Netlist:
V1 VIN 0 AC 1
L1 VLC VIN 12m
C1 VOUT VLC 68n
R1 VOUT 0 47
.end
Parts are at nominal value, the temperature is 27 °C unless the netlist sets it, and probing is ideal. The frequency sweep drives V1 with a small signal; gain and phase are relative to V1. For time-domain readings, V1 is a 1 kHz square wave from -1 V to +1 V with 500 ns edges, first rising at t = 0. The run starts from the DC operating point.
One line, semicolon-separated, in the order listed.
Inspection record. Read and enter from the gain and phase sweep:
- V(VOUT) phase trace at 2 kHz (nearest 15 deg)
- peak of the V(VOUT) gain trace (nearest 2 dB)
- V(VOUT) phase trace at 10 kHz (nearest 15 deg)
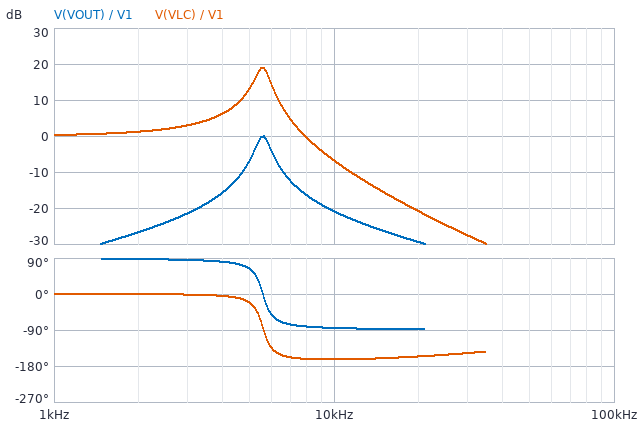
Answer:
90 deg; 0 dB; -90 deg
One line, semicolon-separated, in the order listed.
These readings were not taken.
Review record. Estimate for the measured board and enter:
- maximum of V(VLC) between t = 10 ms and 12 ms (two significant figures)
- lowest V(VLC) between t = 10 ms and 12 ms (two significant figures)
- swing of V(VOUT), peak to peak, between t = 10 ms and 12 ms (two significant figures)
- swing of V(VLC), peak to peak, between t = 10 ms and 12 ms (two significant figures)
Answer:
2.5 V; -2.5 V; 370 mV; 5.0 V
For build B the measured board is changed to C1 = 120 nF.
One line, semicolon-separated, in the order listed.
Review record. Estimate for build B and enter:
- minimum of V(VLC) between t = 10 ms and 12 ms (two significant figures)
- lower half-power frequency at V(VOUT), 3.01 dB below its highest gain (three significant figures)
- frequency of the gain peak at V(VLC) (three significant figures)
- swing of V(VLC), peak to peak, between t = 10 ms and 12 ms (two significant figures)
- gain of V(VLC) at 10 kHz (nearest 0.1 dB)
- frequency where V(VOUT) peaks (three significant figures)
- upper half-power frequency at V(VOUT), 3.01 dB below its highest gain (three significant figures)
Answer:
-2.2 V; 3.89 kHz; 4.17 kHz; 4.4 V; -12.9 dB; 4.19 kHz; 4.52 kHz
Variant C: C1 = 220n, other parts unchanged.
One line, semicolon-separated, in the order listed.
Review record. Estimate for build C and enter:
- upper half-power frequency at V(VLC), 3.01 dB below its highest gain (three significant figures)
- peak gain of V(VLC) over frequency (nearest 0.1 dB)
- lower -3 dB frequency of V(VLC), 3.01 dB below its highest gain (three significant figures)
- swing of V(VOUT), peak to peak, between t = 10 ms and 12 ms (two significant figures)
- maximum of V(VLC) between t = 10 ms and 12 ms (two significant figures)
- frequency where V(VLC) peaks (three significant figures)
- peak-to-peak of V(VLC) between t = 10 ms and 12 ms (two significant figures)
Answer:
3.37 kHz; 14.1 dB; 2.74 kHz; 1.1 V; 3.3 V; 3.07 kHz; 6.7 V
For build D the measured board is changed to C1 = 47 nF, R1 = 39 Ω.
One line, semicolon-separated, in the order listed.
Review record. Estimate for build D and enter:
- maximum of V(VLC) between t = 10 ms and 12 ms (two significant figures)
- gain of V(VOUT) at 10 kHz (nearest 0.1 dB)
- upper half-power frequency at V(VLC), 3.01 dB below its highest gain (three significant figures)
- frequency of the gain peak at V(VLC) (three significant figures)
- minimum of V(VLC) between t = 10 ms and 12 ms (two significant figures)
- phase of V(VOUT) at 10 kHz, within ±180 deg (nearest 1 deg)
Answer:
3.1 V; -20.6 dB; 6.95 kHz; 6.69 kHz; -3.1 V; -85 deg
